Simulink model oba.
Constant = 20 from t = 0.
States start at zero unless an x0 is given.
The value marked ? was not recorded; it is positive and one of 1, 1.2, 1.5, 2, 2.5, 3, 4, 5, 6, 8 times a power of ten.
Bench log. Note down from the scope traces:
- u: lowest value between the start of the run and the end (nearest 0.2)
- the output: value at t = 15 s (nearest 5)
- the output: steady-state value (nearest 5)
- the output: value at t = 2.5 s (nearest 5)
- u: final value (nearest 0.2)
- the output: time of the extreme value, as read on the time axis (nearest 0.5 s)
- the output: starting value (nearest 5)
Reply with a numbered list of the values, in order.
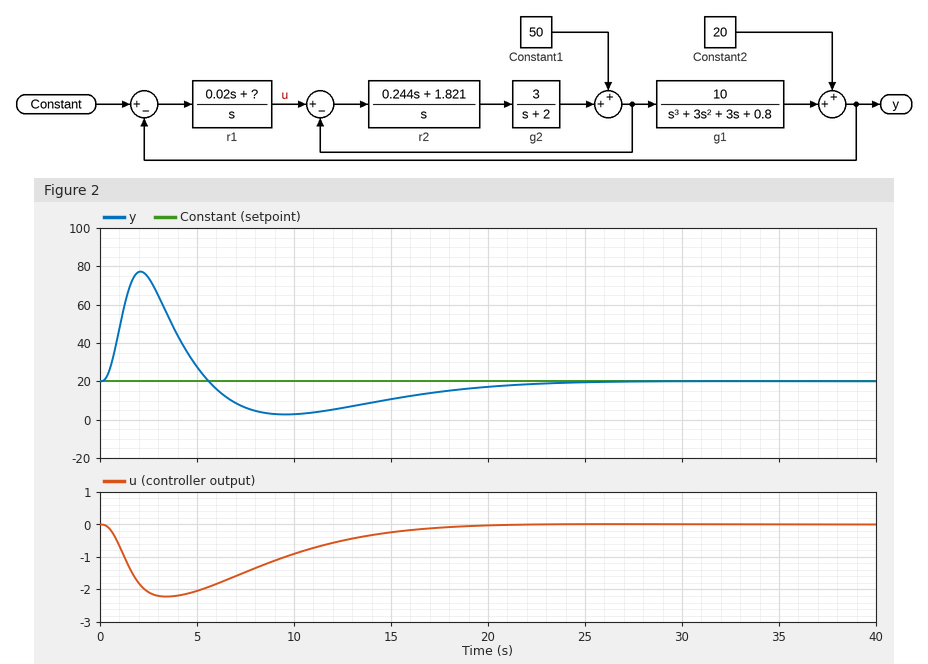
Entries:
1. -2.2
2. 10
3. 20
4. 75
5. 0.0
6. 2.0 s
7. 20
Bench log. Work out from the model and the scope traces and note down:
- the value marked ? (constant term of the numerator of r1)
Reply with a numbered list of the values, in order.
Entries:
1. 0.012
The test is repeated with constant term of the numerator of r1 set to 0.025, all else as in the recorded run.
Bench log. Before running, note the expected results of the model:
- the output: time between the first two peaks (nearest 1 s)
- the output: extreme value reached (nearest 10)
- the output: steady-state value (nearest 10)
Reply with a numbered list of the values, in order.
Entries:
1. 16 s
2. 80
3. 20
